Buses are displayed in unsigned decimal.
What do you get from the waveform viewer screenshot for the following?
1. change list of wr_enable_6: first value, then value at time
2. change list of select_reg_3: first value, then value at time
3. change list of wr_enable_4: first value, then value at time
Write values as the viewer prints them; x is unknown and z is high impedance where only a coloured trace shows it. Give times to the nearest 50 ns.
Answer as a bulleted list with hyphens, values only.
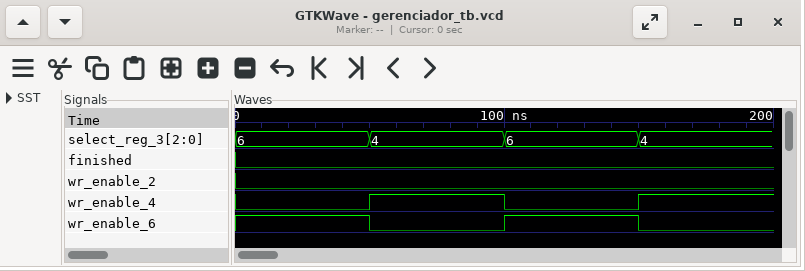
- 1, 0 at 50 ns, 1 at 100 ns, 0 at 150 ns
- 6, 4 at 50 ns, 6 at 100 ns, 4 at 150 ns
- 0, 1 at 50 ns, 0 at 100 ns, 1 at 150 ns
